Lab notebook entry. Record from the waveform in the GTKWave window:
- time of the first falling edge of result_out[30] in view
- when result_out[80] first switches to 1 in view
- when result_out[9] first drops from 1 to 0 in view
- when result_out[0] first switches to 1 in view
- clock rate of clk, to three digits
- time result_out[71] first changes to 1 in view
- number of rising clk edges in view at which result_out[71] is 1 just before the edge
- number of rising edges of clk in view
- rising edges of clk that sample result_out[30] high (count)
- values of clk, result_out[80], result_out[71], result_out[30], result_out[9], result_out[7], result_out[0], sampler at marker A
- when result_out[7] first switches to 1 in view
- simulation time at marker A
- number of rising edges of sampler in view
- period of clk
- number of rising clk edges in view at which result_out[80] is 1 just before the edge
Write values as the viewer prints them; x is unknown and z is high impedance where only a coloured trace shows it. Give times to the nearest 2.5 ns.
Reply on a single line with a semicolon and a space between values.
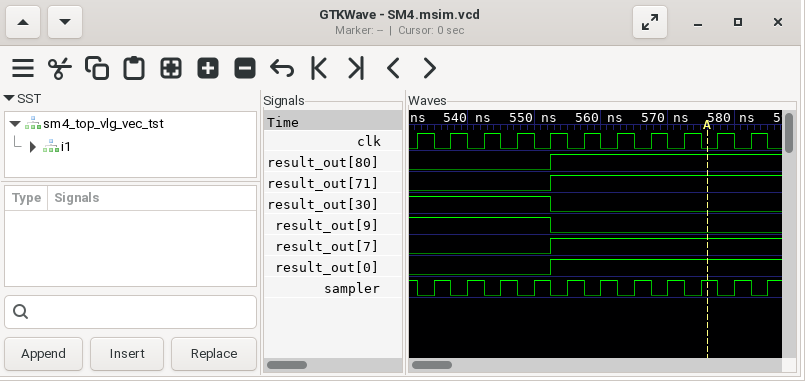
552.5 ns; 552.5 ns; 552.5 ns; 552.5 ns; 200 MHz; 552.5 ns; 6; 11; 5; clk=0, result_out[80]=1, result_out[71]=1, result_out[30]=0, result_out[9]=0, result_out[7]=1, result_out[0]=1, sampler=1; 552.5 ns; 575 ns; 11; 5 ns; 6
